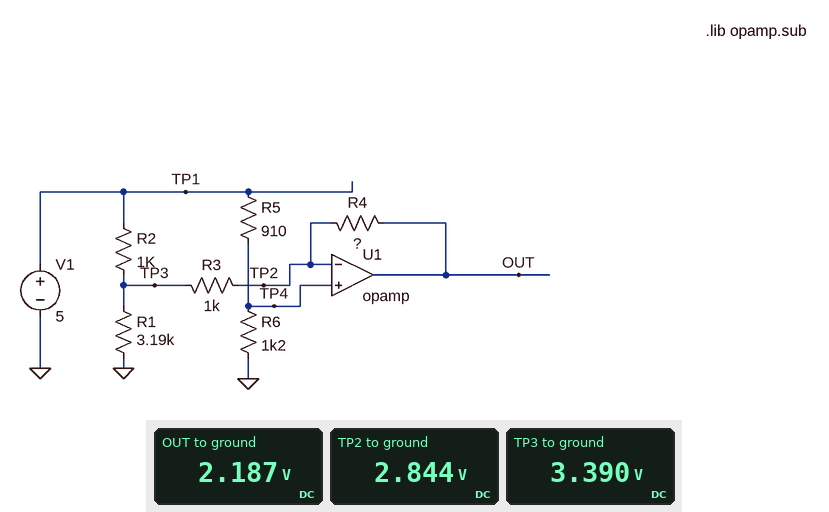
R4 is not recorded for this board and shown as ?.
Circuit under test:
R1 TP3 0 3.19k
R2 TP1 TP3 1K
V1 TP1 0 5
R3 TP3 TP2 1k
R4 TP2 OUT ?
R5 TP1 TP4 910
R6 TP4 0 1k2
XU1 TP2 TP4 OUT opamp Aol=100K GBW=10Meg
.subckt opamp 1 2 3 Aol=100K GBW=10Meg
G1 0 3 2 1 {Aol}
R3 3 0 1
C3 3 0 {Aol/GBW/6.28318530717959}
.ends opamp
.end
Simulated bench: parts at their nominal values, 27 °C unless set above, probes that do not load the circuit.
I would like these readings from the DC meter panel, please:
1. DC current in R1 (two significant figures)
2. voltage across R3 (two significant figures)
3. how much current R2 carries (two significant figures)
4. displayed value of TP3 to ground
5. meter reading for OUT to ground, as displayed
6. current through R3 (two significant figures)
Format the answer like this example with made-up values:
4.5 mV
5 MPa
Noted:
1.1 mA
550 mV
1.6 mA
3.390 V
2.187 V
550 µA
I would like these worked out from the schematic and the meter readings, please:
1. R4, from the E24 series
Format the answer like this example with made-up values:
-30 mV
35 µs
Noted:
1.2 kΩ
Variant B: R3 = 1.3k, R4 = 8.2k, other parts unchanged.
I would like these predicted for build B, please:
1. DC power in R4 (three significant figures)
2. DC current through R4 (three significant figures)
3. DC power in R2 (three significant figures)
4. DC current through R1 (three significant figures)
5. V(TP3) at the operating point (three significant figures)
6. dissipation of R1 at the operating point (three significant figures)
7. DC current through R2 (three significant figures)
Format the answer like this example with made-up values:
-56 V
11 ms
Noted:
1.79 mW
467 µA
2.40 mW
1.08 mA
3.45 V
3.73 mW
1.55 mA
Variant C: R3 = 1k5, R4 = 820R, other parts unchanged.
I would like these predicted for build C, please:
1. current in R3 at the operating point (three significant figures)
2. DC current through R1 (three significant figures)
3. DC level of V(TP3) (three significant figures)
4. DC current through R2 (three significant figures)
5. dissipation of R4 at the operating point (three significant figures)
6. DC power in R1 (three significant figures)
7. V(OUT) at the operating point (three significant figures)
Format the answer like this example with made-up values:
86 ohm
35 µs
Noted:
426 µA
1.09 mA
3.48 V
1.52 mA
149 µW
3.80 mW
2.49 V
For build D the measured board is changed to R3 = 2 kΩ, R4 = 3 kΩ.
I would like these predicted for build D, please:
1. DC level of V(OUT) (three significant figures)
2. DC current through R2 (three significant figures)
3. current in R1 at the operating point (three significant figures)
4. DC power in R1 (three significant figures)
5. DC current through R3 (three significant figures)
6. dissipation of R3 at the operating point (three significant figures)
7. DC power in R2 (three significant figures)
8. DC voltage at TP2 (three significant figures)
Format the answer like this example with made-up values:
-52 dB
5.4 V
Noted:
1.80 V
1.46 mA
1.11 mA
3.93 mW
349 µA
243 µW
2.13 mW
2.84 V
